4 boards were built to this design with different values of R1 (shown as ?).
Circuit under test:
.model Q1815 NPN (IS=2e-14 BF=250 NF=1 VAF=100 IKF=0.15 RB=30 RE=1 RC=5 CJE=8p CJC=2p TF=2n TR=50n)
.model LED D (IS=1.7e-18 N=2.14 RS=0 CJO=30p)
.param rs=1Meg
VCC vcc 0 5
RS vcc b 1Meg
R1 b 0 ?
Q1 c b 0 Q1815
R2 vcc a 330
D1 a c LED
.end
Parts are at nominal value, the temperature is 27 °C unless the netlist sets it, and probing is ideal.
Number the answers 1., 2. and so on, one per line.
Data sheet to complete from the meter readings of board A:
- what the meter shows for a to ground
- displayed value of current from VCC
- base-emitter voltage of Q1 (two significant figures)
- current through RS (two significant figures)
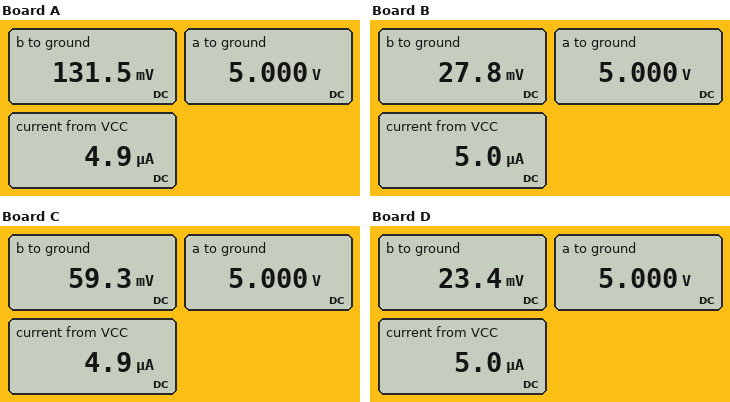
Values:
1. 5.000 V
2. 4.9 µA
3. 130 mV
4. 4.9 µA
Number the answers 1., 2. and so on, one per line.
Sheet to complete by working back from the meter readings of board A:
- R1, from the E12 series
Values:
1. 27 kΩ
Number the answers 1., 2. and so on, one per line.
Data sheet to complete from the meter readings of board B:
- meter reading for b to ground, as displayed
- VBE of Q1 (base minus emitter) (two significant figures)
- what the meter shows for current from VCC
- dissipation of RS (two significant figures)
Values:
1. 27.8 mV
2. 28 mV
3. 5.0 µA
4. 25 µW
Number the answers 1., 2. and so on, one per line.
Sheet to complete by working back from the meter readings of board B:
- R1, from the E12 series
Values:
1. 5.6 kΩ
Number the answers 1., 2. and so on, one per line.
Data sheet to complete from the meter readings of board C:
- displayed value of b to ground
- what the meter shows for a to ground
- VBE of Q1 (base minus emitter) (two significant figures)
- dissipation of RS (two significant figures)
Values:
1. 59.3 mV
2. 5.000 V
3. 59 mV
4. 24 µW
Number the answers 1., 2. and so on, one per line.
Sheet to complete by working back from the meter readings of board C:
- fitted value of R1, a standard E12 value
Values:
1. 12 kΩ
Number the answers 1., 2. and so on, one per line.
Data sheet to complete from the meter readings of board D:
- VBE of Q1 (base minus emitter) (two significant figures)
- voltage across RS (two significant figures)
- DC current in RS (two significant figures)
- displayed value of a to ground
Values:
1. 23 mV
2. 5.0 V
3. 5.0 µA
4. 5.000 V
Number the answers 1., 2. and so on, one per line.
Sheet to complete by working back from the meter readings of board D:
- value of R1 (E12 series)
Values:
1. 4.7 kΩ
